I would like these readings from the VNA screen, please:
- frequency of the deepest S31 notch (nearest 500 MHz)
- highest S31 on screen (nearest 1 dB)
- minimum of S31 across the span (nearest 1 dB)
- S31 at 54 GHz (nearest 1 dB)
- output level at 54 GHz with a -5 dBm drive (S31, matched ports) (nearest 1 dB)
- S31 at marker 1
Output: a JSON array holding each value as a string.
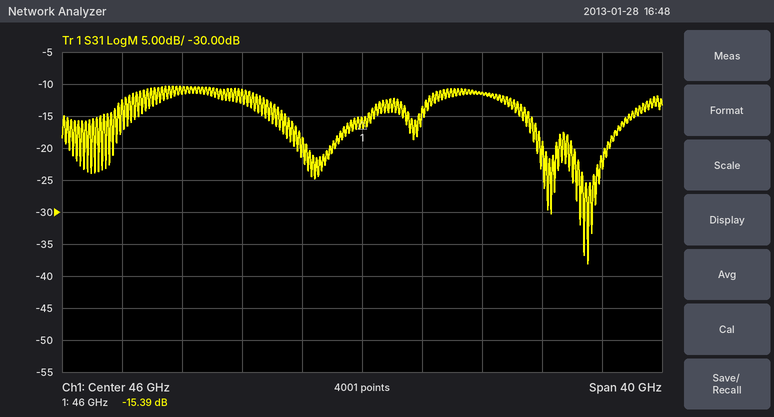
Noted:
["61.0 GHz", "-10 dB", "-38 dB", "-11 dB", "-16 dBm", "-15.39 dB"]
